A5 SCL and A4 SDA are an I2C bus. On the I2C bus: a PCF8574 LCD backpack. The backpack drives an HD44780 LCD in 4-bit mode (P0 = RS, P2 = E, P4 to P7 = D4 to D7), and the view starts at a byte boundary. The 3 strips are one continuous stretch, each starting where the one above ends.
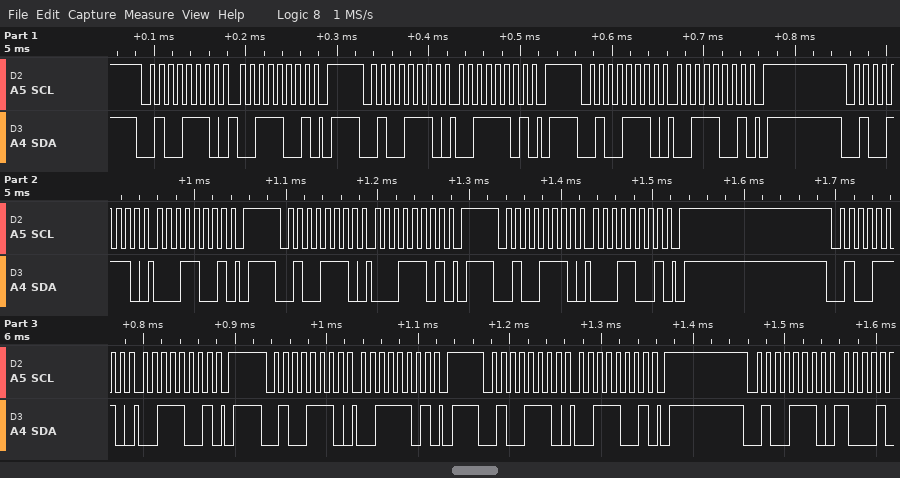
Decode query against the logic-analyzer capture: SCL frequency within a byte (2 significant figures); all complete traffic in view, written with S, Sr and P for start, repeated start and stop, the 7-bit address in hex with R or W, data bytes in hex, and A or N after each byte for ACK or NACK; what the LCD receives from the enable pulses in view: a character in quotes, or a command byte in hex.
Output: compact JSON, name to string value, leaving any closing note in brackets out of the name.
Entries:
{"SCL frequency within a byte": "100 kHz", "all complete traffic in view, written with S, Sr and P for start, repeated start and stop, the 7-bit address in hex with R or W, data bytes in hex, and A or N after each byte for ACK or NACK": "S 27W A 39 A P S 27W A 3D A P S 27W A 39 A P S 27W A 19 A P S 27W A 1D A P S 27W A 19 A P S 27W A 39 A P S 27W A 3D A P S 27W A 39 A P S 27W A", "what the LCD receives from the enable pulses in view: a character in quotes, or a command byte in hex": "'1'"}
